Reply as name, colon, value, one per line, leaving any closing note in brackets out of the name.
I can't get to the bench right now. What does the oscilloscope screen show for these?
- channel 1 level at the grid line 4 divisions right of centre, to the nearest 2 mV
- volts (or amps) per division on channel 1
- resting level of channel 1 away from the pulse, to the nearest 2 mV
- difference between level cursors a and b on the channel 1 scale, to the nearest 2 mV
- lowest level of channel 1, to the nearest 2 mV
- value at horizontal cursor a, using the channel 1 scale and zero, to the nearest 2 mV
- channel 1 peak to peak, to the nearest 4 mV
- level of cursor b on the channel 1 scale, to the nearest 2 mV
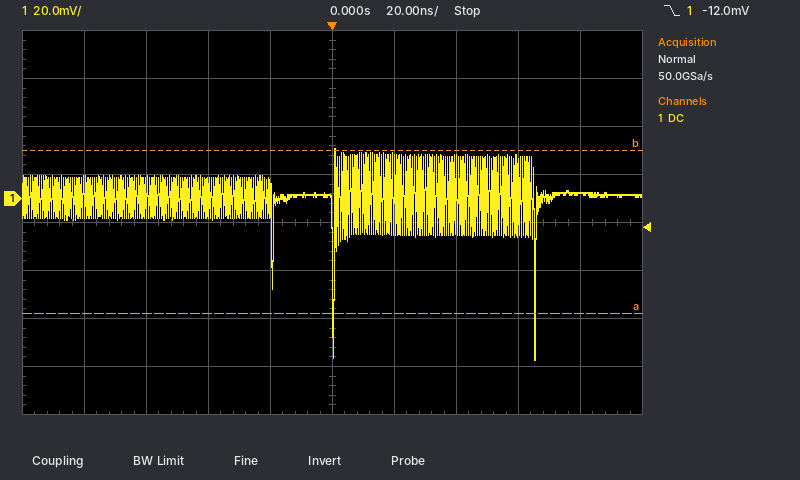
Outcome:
channel 1 level at the grid line 4 divisions right of centre, to the nearest 2 mV: 2 mV
volts (or amps) per division on channel 1: 20 mV
resting level of channel 1 away from the pulse, to the nearest 2 mV: 2 mV
difference between level cursors a and b on the channel 1 scale, to the nearest 2 mV: 68 mV
lowest level of channel 1, to the nearest 2 mV: -68 mV
value at horizontal cursor a, using the channel 1 scale and zero, to the nearest 2 mV: -48 mV
channel 1 peak to peak, to the nearest 4 mV: 88 mV
level of cursor b on the channel 1 scale, to the nearest 2 mV: 20 mV
